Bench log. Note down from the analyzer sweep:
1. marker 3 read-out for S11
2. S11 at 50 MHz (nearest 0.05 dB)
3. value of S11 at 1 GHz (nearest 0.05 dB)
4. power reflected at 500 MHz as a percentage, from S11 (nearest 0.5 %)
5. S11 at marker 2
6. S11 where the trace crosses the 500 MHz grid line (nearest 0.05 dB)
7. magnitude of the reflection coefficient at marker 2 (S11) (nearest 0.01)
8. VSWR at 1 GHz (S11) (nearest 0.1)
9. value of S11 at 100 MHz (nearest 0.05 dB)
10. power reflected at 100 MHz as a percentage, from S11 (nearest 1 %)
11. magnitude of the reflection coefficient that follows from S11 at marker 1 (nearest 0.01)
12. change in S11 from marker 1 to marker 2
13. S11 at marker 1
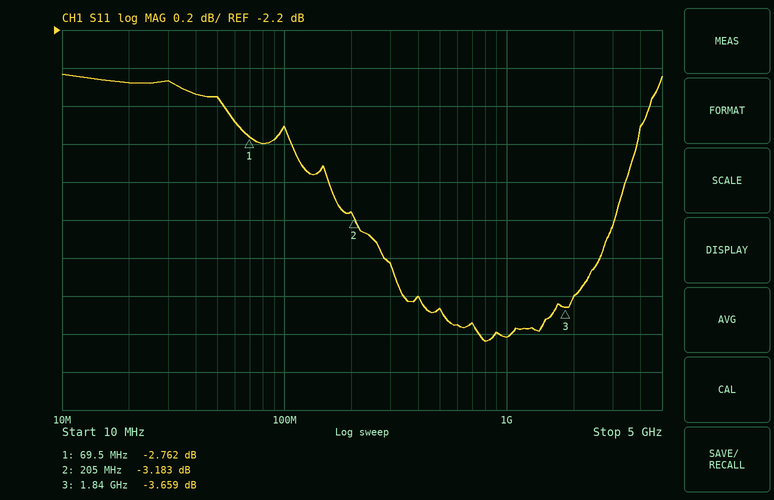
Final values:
-3.659 dB
-2.55 dB
-3.80 dB
43.0 %
-3.183 dB
-3.65 dB
0.69
4.6
-2.70 dB
54 %
0.73
-0.421 dB
-2.762 dB
